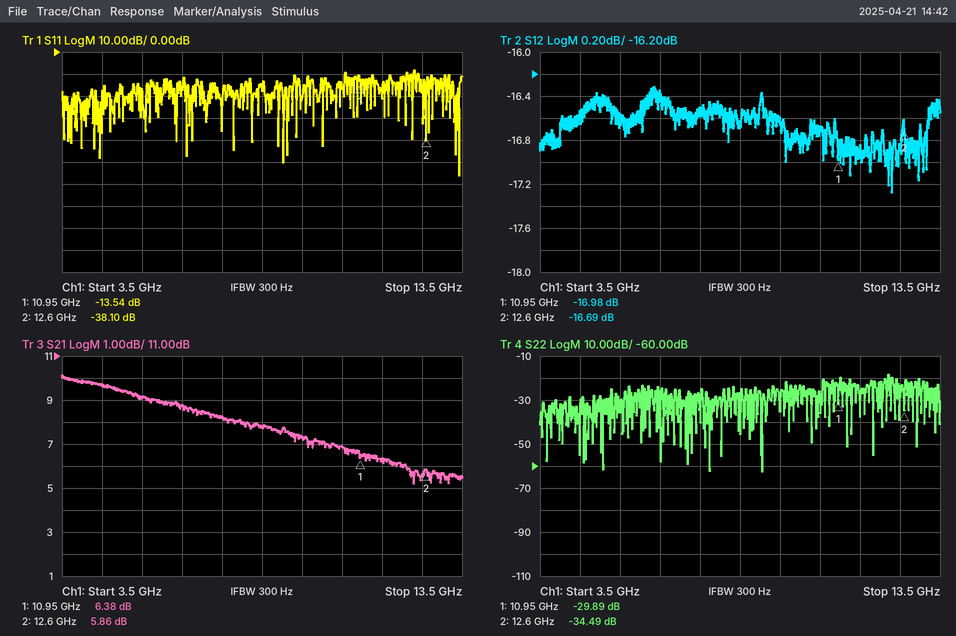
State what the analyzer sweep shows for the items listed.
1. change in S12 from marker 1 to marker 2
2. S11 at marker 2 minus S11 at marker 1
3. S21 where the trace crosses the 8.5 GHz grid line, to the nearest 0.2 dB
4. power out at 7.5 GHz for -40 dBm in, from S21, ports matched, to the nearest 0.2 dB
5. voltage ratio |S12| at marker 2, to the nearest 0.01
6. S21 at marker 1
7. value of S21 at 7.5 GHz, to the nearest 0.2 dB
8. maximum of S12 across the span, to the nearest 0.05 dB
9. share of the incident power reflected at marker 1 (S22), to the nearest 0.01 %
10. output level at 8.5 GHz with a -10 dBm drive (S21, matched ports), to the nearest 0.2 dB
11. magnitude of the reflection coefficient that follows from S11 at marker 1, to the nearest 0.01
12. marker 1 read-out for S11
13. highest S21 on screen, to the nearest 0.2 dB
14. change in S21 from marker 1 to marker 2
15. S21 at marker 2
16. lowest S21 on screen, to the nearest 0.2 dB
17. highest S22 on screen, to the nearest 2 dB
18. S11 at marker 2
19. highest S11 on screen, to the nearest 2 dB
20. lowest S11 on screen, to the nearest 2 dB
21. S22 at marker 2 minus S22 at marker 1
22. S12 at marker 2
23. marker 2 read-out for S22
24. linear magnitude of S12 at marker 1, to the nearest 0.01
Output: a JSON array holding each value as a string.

["0.29 dB", "-24.56 dB", "7.8 dB", "-31.8 dBm", "0.15", "6.38 dB", "8.2 dB", "-16.30 dB", "0.10 %", "-2.2 dBm", "0.21", "-13.54 dB", "10.2 dB", "-0.52 dB", "5.86 dB", "5.2 dB", "-18 dB", "-38.10 dB", "-8 dB", "-56 dB", "-4.60 dB", "-16.69 dB", "-34.49 dB", "0.14"]
